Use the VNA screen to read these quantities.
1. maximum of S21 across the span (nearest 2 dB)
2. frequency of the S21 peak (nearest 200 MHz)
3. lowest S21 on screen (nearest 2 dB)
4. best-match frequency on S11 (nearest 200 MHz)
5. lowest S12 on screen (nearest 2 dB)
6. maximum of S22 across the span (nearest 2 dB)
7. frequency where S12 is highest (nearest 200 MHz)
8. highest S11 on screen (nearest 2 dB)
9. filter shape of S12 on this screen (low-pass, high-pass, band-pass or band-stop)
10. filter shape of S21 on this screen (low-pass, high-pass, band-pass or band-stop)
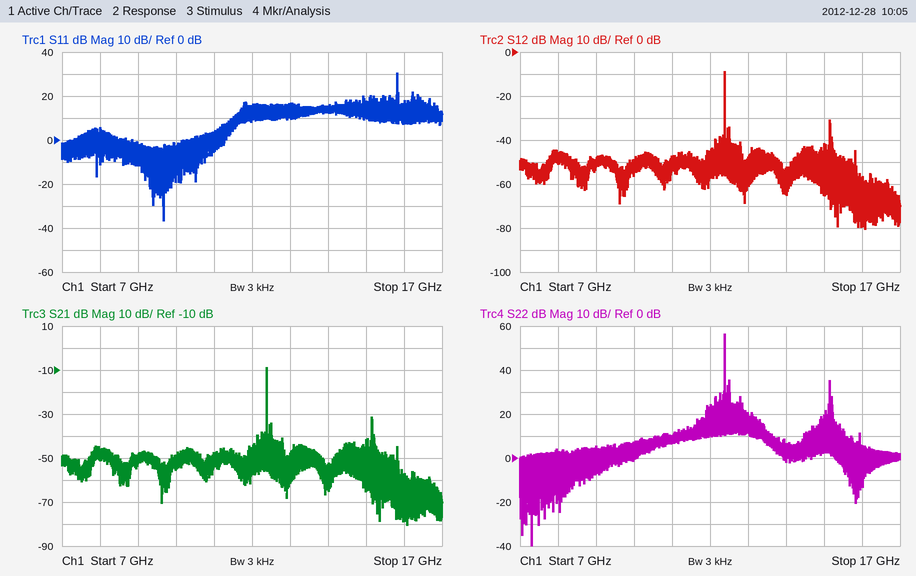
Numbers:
-8 dB
12.4 GHz
-80 dB
9.6 GHz
-80 dB
56 dB
12.4 GHz
30 dB
band-pass
band-pass
